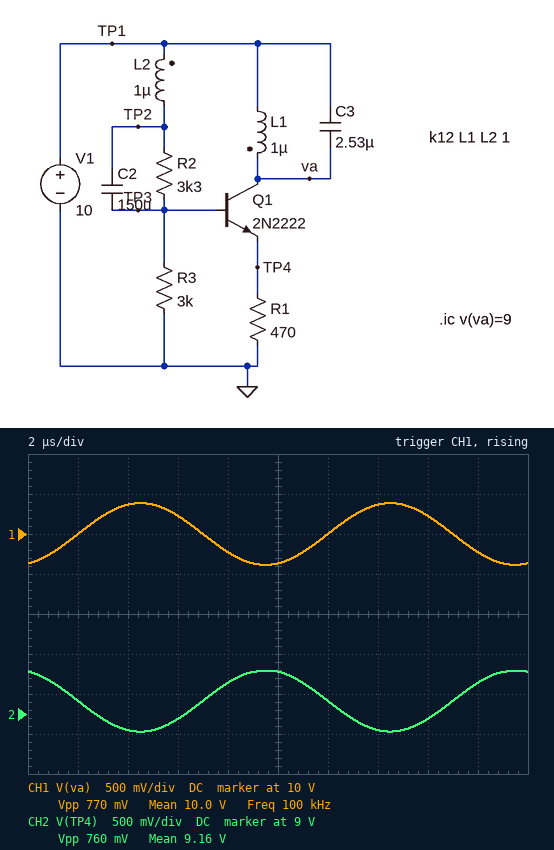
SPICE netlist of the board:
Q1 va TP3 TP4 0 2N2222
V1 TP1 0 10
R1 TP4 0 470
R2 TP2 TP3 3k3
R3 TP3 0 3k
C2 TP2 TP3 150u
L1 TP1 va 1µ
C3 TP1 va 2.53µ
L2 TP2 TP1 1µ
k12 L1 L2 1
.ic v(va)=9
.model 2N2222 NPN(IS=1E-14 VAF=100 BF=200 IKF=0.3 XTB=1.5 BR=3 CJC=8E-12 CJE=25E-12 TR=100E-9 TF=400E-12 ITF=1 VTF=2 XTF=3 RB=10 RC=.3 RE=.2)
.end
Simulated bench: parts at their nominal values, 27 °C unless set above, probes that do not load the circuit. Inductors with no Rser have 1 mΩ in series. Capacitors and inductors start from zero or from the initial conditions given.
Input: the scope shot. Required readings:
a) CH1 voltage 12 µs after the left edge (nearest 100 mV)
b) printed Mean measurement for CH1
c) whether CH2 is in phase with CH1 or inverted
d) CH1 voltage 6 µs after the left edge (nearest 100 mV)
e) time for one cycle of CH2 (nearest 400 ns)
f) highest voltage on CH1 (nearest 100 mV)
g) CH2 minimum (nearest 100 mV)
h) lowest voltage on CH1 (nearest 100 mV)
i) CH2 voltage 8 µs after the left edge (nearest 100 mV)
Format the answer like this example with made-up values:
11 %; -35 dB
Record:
10.0 V; 10.0 V; inverted; 10.2 V; 10.0 µs; 10.4 V; 8.8 V; 9.6 V; 9.4 V
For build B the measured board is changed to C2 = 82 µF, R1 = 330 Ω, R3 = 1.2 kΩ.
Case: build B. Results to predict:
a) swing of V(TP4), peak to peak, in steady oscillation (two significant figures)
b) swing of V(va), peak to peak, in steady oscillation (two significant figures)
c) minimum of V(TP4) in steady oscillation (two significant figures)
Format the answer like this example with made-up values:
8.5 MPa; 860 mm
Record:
870 mV; 880 mV; 8.6 V
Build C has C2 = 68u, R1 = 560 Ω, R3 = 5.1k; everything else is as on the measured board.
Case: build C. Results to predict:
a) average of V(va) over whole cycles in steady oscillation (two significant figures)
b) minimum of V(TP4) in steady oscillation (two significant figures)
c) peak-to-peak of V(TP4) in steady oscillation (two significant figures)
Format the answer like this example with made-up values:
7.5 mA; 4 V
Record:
10 V; 8.6 V; 860 mV
